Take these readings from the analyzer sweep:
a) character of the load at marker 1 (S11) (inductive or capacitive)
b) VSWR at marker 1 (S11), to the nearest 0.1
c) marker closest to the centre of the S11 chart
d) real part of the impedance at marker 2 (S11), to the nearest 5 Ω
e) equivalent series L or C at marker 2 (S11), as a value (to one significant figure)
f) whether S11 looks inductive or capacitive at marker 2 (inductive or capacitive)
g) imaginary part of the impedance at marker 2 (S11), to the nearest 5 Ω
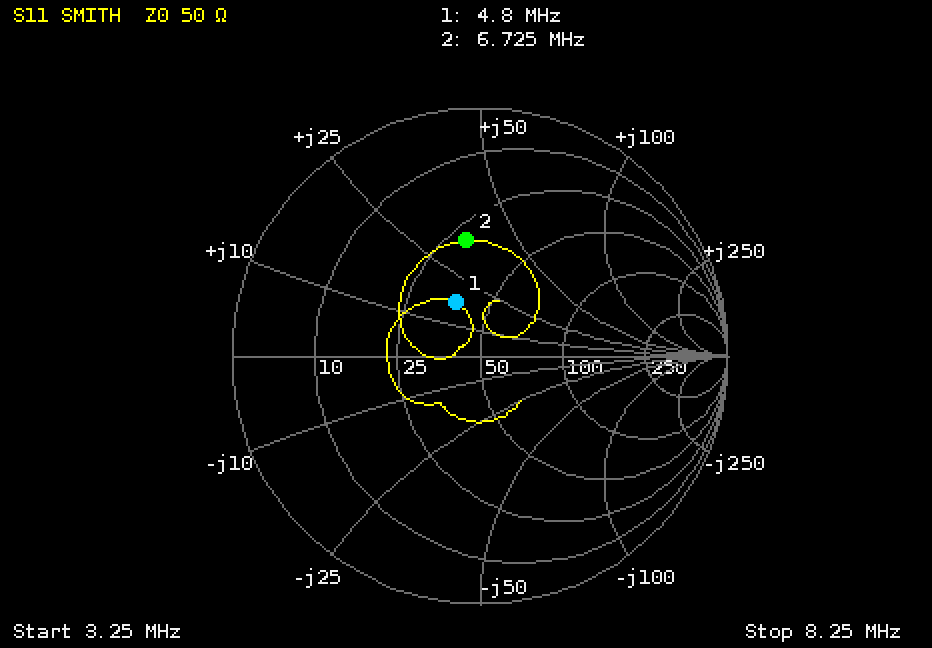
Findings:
inductive
1.6
marker 1
30 Ω
800 nH
inductive
+35 Ω
